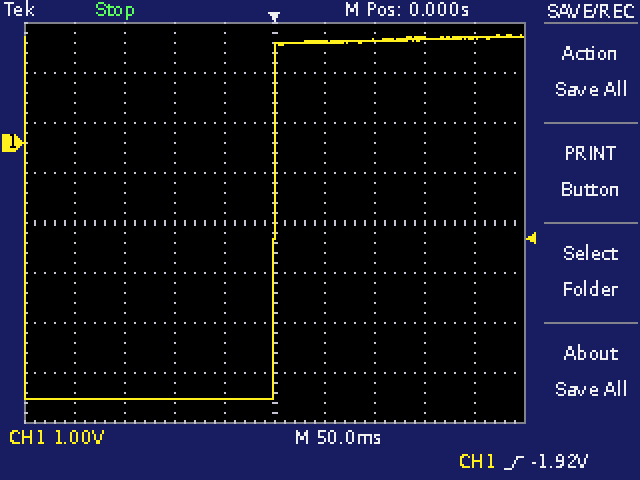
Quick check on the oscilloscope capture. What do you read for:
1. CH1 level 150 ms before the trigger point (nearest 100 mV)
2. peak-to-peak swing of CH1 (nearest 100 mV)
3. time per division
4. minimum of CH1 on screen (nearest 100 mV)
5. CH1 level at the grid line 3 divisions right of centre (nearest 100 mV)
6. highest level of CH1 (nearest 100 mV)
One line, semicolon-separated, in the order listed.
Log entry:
-5.1 V; 7.3 V; 50 ms; -5.1 V; 2.1 V; 2.2 V
